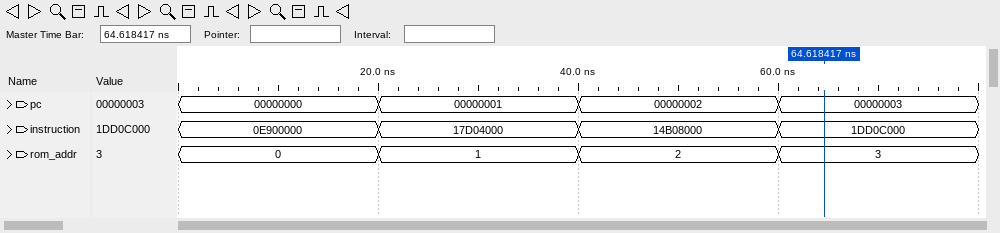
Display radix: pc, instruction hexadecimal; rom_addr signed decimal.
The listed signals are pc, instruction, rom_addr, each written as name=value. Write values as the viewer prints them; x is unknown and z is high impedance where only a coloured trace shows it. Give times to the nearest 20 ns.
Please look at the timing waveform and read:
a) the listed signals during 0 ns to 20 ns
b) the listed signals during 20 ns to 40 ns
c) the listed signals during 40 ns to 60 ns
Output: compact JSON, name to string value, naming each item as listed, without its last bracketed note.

{"the listed signals during 0 ns to 20 ns": "pc=00000000, instruction=0E900000, rom_addr=0", "the listed signals during 20 ns to 40 ns": "pc=00000001, instruction=17D04000, rom_addr=1", "the listed signals during 40 ns to 60 ns": "pc=00000002, instruction=14B08000, rom_addr=2"}
